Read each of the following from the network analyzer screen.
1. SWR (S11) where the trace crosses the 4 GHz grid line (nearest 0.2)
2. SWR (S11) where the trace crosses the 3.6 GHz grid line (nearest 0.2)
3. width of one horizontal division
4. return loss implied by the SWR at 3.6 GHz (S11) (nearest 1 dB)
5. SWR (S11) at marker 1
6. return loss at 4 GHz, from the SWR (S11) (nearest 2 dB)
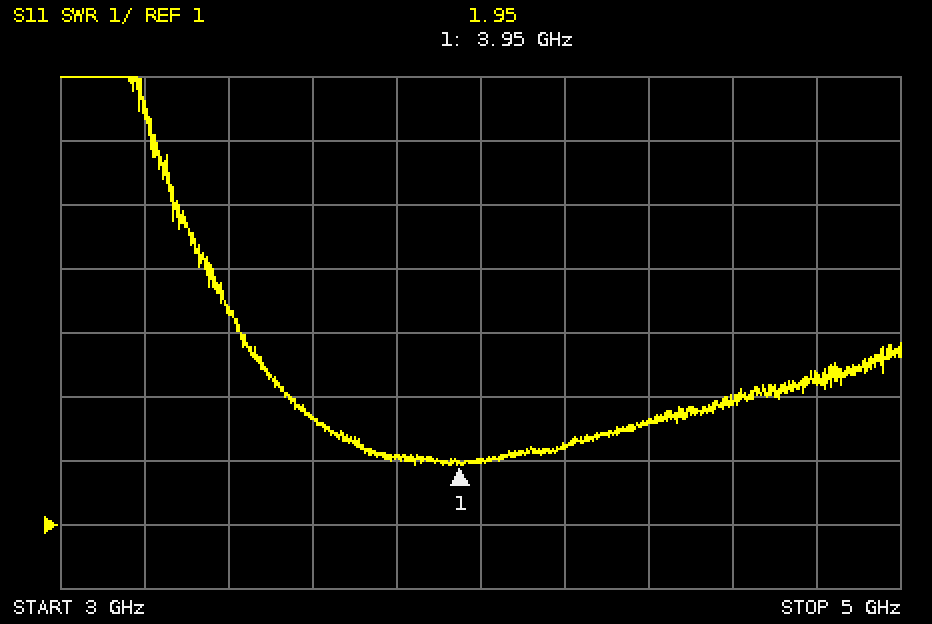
2.0
2.6
200 MHz
7 dB
1.95
10 dB
